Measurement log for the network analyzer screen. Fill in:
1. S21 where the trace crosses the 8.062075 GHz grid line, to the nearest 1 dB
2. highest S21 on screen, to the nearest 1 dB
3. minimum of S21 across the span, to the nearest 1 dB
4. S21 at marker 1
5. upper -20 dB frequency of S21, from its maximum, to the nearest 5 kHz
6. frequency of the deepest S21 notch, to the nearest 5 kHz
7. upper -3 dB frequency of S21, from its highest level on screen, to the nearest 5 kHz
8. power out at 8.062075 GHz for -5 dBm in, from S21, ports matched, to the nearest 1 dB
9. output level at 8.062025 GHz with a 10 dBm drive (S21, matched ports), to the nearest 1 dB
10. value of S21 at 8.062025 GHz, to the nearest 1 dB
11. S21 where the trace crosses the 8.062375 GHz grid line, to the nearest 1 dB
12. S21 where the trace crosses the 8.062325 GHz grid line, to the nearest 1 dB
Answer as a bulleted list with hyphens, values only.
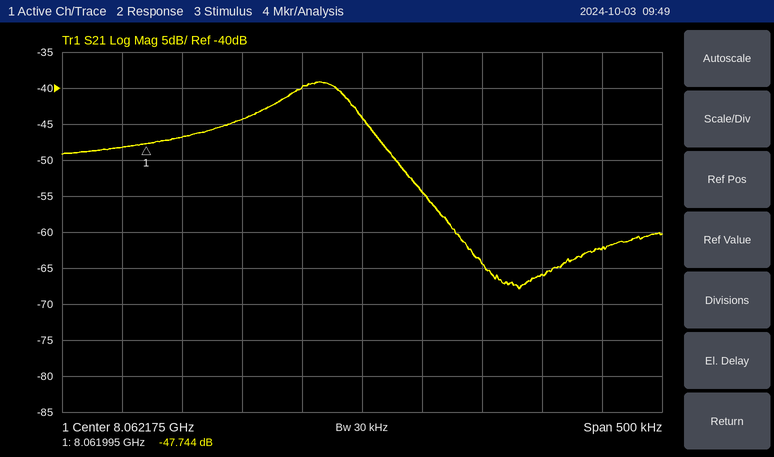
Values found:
- -44 dB
- -39 dB
- -68 dB
- -47.744 dB
- 8.062250 GHz
- 8.062305 GHz
- 8.062165 GHz
- -49 dBm
- -37 dBm
- -47 dB
- -62 dB
- -66 dB
